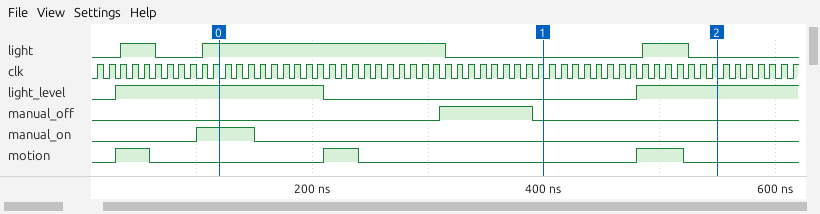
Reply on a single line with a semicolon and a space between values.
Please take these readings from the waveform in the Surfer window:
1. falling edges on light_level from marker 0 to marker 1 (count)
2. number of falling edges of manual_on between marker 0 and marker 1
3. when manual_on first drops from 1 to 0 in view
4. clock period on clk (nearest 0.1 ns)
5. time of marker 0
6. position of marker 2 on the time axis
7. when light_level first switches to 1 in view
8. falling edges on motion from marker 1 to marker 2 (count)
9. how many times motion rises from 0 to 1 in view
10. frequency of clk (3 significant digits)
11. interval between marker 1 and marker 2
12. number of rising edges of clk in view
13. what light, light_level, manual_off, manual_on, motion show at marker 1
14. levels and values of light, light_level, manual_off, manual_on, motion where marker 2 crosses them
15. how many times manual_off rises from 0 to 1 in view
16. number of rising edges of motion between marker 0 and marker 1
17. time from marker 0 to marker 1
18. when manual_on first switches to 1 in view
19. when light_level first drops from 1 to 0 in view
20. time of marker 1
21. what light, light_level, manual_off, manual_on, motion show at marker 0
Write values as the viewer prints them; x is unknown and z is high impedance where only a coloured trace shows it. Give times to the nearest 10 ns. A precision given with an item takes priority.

1; 1; 150 ns; 10 ns; 120 ns; 550 ns; 30 ns; 1; 3; 100 MHz; 150 ns; 61; light=0, light_level=0, manual_off=0, manual_on=0, motion=0; light=0, light_level=1, manual_off=0, manual_on=0, motion=0; 1; 1; 280 ns; 100 ns; 210 ns; 400 ns; light=1, light_level=1, manual_off=0, manual_on=1, motion=0
